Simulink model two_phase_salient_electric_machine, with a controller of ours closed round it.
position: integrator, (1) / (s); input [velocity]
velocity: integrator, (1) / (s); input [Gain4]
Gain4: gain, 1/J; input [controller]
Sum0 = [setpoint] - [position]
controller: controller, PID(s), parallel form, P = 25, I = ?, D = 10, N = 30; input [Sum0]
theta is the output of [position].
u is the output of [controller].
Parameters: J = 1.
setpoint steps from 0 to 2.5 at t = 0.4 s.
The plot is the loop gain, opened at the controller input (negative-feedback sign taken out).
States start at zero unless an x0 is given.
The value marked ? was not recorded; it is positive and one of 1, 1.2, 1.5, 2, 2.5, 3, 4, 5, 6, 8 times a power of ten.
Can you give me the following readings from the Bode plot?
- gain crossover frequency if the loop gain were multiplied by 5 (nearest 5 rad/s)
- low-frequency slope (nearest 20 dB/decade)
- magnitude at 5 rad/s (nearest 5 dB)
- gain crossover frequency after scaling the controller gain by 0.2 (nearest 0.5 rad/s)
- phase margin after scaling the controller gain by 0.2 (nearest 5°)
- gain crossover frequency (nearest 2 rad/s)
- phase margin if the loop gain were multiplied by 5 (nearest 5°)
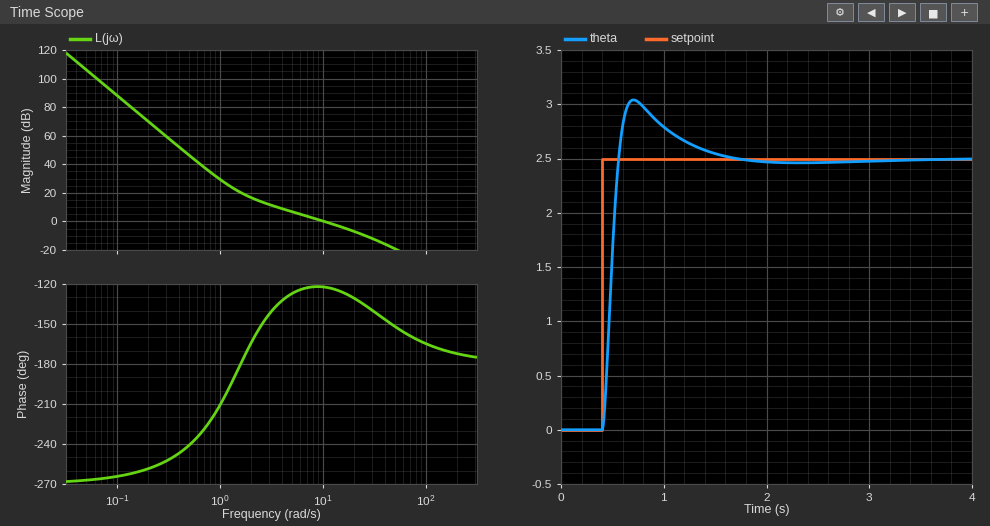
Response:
35 rad/s
-60 dB/decade
5 dB
2.5 rad/s
30°
10 rad/s
35°
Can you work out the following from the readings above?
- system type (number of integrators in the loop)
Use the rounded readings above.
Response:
3
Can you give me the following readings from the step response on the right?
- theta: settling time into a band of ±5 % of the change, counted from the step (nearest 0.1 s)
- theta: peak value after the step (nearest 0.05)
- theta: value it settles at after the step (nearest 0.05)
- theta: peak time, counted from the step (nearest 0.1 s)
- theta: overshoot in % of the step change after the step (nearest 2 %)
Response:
0.9 s
3.05
2.50
0.3 s
22 %
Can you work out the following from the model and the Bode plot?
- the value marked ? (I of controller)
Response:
25
